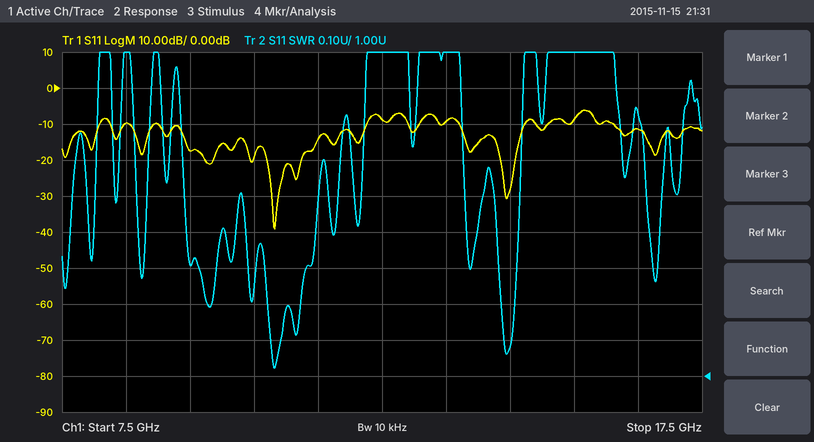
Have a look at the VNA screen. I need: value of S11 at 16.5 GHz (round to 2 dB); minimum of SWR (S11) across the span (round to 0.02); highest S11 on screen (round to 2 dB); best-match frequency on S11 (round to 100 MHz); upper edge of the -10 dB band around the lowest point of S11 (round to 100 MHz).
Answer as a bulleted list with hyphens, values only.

- -12 dB
- 1.02
- -6 dB
- 10.8 GHz
- 12.3 GHz
